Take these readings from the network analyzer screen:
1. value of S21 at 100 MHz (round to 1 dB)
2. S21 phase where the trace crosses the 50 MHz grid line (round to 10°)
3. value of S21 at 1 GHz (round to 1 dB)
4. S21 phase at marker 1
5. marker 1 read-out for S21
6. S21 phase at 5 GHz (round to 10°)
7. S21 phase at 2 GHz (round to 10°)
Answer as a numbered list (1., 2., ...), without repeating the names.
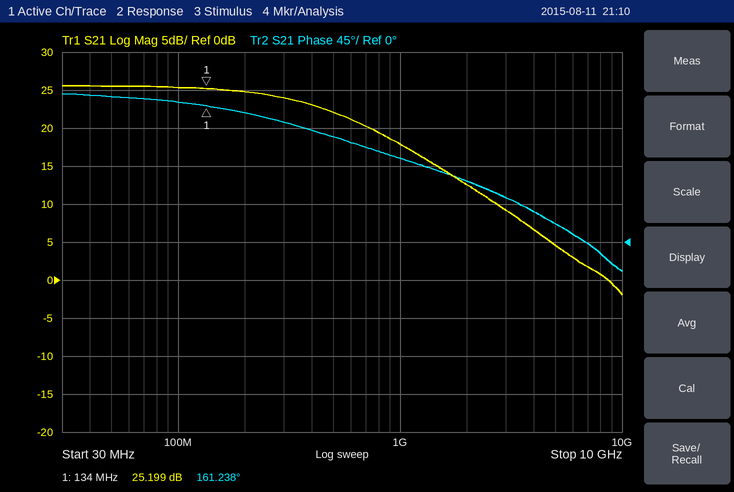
1. 25 dB
2. 170°
3. 18 dB
4. 161.238°
5. 25.199 dB
6. 20°
7. 70°
